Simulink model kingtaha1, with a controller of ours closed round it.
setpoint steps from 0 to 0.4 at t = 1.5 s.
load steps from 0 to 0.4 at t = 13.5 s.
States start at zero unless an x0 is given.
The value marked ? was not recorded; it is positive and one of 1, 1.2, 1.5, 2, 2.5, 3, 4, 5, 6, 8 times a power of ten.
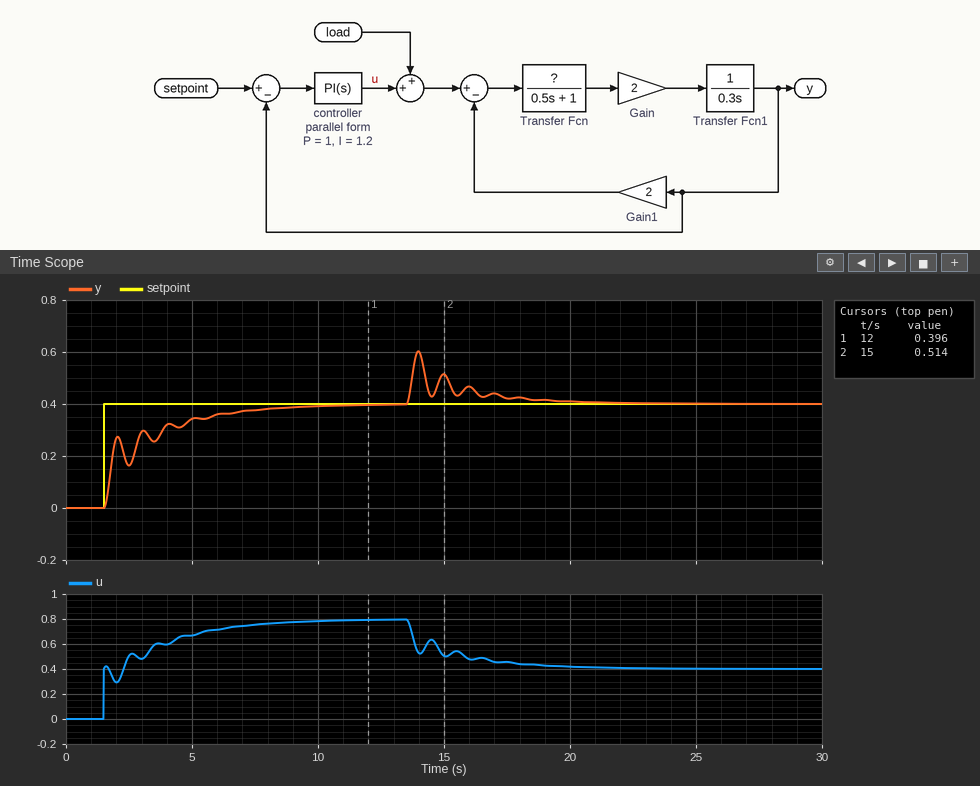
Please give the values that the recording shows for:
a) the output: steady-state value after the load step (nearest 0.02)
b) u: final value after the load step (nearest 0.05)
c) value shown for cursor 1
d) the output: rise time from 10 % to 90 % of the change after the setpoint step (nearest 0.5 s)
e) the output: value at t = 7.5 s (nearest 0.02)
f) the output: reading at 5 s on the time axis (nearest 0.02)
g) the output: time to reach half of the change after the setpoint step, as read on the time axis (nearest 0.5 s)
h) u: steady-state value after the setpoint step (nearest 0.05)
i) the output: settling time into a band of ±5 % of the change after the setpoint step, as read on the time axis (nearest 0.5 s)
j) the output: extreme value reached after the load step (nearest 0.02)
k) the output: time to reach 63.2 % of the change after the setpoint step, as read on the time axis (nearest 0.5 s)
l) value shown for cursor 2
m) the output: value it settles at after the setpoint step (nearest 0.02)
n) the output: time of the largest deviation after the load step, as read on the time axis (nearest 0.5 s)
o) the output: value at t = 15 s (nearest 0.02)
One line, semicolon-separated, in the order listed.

0.40; 0.40; 0.396; 4.5 s; 0.38; 0.34; 2.0 s; 0.80; 8.0 s; 0.60; 2.0 s; 0.514; 0.40; 14.0 s; 0.52
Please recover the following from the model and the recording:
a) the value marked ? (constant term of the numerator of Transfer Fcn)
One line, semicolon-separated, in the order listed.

1
